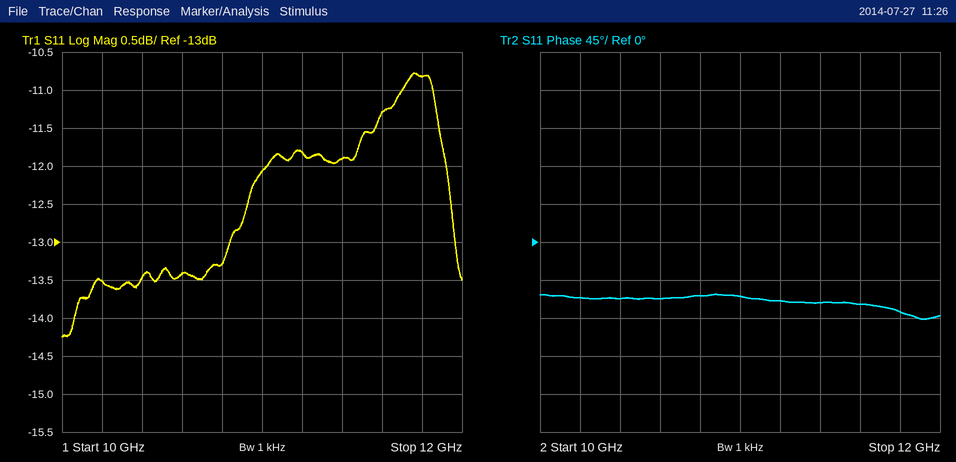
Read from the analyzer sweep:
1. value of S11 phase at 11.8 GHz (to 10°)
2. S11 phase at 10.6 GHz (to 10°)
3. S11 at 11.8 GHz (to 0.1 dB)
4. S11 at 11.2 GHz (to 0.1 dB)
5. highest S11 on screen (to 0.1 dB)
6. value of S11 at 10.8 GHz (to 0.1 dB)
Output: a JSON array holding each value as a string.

["-80°", "-70°", "-10.8 dB", "-11.8 dB", "-10.8 dB", "-13.3 dB"]
